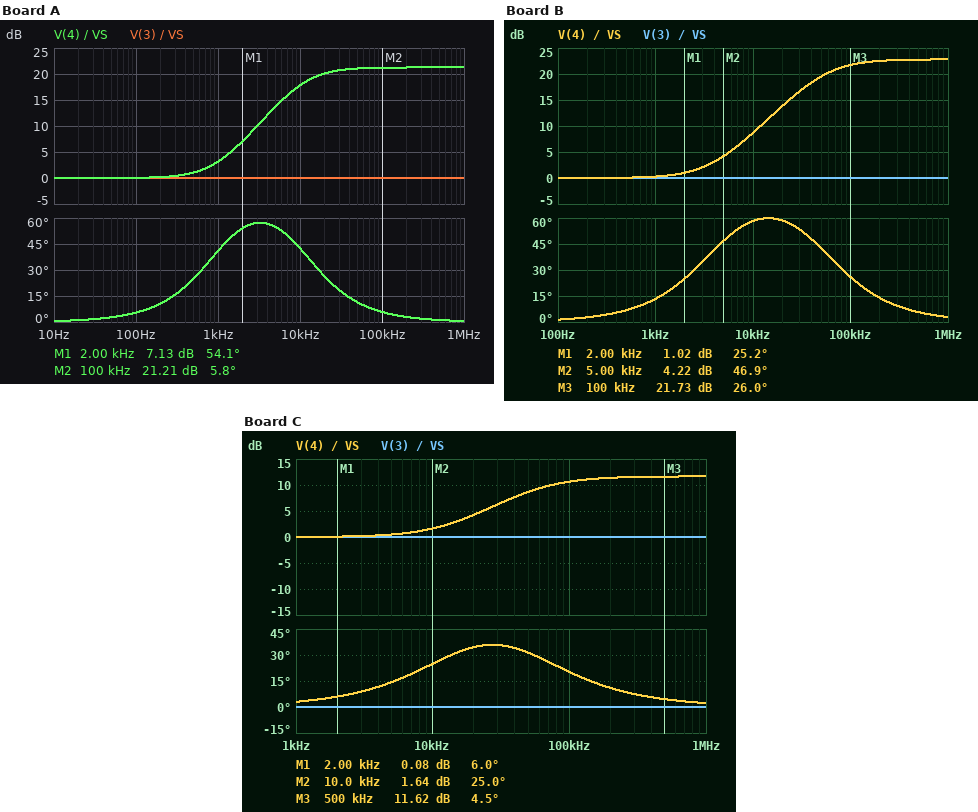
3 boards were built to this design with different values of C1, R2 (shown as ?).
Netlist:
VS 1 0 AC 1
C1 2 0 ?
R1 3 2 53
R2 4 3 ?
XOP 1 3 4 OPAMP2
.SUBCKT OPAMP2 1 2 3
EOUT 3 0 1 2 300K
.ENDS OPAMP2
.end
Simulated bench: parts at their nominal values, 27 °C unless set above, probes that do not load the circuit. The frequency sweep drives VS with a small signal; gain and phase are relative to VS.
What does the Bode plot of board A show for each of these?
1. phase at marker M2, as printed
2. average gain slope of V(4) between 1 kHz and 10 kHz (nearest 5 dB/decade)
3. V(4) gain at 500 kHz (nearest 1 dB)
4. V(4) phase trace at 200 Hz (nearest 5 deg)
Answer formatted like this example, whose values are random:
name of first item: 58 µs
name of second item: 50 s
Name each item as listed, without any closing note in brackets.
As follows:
phase at marker M2, as printed: 5.8 deg
average gain slope of V(4) between 1 kHz and 10 kHz: 15 dB/decade
V(4) gain at 500 kHz: 21 dB
V(4) phase trace at 200 Hz: 10 deg
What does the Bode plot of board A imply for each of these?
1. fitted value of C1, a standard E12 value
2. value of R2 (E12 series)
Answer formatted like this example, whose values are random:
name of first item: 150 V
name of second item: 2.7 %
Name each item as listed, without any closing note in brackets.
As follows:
fitted value of C1, a standard E12 value: 270 nF
value of R2: 560 Ω
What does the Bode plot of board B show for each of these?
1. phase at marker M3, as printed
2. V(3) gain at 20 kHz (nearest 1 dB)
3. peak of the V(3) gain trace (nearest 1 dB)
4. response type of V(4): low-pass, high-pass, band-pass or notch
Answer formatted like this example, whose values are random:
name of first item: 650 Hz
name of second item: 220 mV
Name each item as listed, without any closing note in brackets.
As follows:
phase at marker M3, as printed: 26.0 deg
V(3) gain at 20 kHz: 0 dB
peak of the V(3) gain trace: 0 dB
response type of V(4): low-pass, high-pass, band-pass or notch: high-pass
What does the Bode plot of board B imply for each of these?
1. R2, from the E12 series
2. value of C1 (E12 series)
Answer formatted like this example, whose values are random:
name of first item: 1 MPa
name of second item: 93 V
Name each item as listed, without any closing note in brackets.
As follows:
R2, from the E12 series: 680 Ω
value of C1: 56 nF
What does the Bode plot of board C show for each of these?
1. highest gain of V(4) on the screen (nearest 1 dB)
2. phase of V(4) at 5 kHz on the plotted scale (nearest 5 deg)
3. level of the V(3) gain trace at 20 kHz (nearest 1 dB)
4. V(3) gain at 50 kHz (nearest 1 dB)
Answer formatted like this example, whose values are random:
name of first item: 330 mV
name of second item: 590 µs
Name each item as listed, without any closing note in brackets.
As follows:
highest gain of V(4) on the screen: 12 dB
phase of V(4) at 5 kHz on the plotted scale: 15 deg
level of the V(3) gain trace at 20 kHz: 0 dB
V(3) gain at 50 kHz: 0 dB
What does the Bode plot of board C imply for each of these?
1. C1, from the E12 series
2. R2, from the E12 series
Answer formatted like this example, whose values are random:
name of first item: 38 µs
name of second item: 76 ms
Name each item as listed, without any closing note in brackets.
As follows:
C1, from the E12 series: 56 nF
R2, from the E12 series: 150 Ω
